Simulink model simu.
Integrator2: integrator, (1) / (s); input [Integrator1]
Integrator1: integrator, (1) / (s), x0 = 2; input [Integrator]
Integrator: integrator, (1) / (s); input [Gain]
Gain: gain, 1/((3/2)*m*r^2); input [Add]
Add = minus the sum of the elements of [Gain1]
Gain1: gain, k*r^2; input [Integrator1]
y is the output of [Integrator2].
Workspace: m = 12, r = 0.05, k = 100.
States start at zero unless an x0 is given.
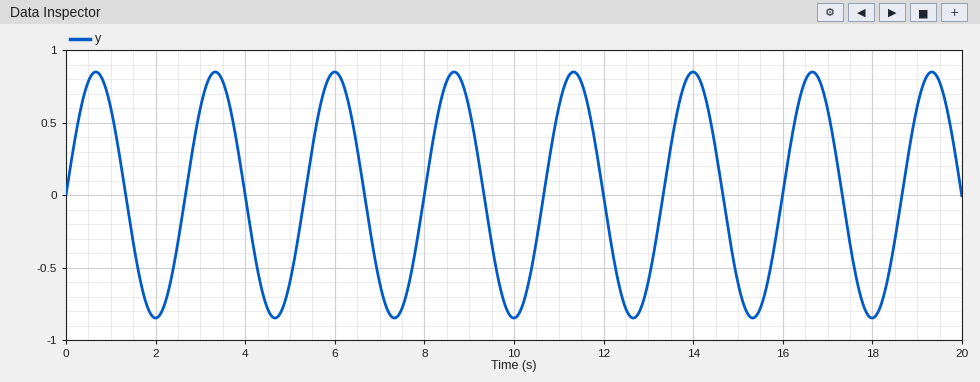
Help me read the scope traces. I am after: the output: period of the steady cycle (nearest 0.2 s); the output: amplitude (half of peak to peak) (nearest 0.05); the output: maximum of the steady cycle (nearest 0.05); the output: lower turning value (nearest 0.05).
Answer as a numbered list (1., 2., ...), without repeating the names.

1. 2.6 s
2. 0.85
3. 0.85
4. -0.85
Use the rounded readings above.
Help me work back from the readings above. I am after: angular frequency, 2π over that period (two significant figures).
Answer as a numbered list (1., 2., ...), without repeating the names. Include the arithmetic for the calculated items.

1. 2π / 2.6 = 2.4 rad/s
